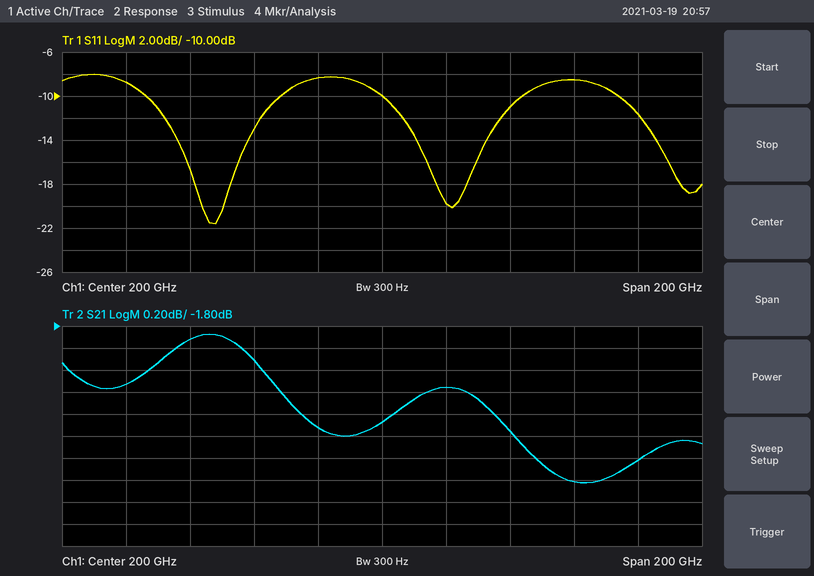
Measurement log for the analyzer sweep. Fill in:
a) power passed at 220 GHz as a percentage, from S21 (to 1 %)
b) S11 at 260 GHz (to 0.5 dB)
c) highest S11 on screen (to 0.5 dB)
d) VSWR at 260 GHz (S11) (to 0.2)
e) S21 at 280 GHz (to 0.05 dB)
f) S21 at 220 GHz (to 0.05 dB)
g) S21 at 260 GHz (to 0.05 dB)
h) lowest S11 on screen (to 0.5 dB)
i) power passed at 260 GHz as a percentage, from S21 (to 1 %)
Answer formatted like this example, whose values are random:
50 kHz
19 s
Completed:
58 %
-8.5 dB
-8.0 dB
2.2
-3.00 dB
-2.35 dB
-3.20 dB
-21.5 dB
48 %
